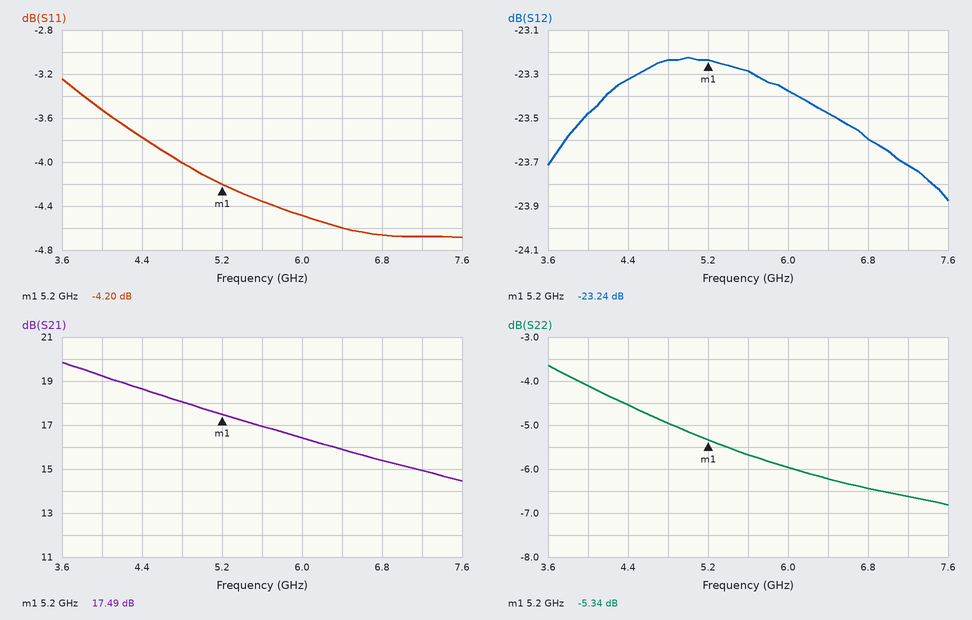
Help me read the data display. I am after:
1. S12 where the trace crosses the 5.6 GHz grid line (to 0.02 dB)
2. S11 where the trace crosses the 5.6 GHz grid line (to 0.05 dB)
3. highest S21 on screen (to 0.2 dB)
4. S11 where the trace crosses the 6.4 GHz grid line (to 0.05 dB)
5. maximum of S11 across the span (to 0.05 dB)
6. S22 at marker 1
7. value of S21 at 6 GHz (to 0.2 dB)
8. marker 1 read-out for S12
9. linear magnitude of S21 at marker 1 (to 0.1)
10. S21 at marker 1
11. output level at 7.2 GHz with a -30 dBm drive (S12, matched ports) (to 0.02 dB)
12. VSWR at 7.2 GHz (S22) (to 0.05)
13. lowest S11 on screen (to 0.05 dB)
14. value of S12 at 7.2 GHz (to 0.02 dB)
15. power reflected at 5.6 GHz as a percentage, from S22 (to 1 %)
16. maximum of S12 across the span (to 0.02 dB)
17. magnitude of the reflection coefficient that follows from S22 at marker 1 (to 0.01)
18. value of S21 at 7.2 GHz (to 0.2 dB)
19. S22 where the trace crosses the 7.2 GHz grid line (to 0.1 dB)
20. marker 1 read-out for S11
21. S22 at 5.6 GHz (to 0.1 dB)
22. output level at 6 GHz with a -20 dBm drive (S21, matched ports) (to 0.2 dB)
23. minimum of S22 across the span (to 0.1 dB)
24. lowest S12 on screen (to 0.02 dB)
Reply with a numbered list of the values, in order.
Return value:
1. -23.28 dB
2. -4.35 dB
3. 19.8 dB
4. -4.60 dB
5. -3.25 dB
6. -5.34 dB
7. 16.4 dB
8. -23.24 dB
9. 7.5
10. 17.49 dB
11. -53.72 dBm
12. 2.75
13. -4.70 dB
14. -23.72 dB
15. 27 %
16. -23.22 dB
17. 0.54
18. 15.0 dB
19. -6.6 dB
20. -4.20 dB
21. -5.7 dB
22. -3.6 dBm
23. -6.8 dB
24. -23.88 dB
